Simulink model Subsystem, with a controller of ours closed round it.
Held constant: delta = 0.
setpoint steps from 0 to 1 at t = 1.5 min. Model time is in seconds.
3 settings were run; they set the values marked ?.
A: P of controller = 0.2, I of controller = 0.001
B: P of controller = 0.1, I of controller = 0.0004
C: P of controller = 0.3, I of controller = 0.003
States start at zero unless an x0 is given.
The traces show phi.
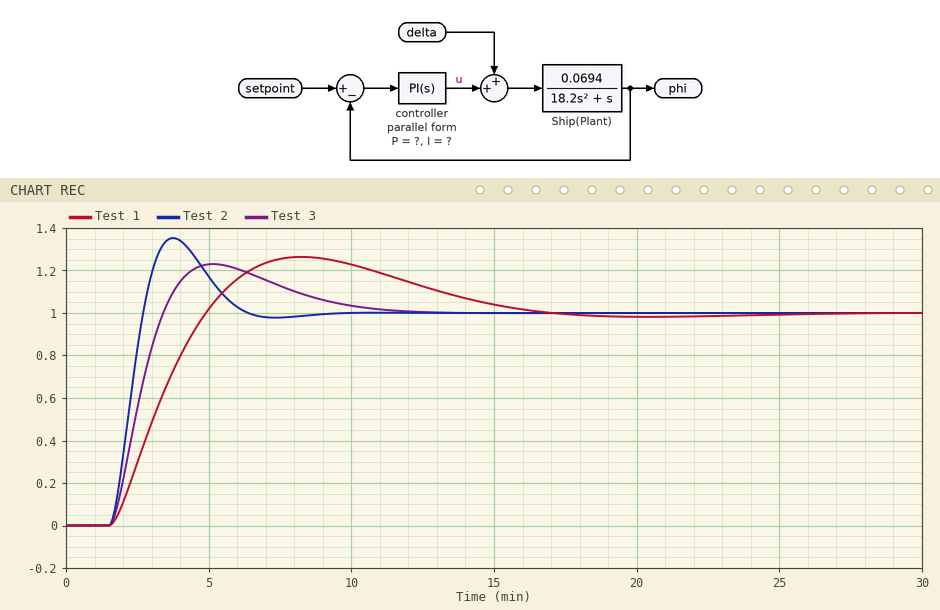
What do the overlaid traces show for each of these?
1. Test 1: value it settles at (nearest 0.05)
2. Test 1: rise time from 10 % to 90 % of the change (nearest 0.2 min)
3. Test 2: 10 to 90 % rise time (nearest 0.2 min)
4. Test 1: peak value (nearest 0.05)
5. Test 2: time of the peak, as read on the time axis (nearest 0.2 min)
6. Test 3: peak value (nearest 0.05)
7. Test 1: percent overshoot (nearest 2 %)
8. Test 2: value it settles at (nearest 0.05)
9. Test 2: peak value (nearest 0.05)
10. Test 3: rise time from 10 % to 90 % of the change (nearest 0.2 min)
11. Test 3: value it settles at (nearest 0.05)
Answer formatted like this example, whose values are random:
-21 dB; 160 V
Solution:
1.00; 2.4 min; 0.8 min; 1.25; 3.8 min; 1.25; 26 %; 1.00; 1.35; 1.4 min; 1.00
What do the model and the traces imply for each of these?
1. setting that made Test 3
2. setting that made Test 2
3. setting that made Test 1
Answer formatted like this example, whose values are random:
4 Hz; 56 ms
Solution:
A; C; B
